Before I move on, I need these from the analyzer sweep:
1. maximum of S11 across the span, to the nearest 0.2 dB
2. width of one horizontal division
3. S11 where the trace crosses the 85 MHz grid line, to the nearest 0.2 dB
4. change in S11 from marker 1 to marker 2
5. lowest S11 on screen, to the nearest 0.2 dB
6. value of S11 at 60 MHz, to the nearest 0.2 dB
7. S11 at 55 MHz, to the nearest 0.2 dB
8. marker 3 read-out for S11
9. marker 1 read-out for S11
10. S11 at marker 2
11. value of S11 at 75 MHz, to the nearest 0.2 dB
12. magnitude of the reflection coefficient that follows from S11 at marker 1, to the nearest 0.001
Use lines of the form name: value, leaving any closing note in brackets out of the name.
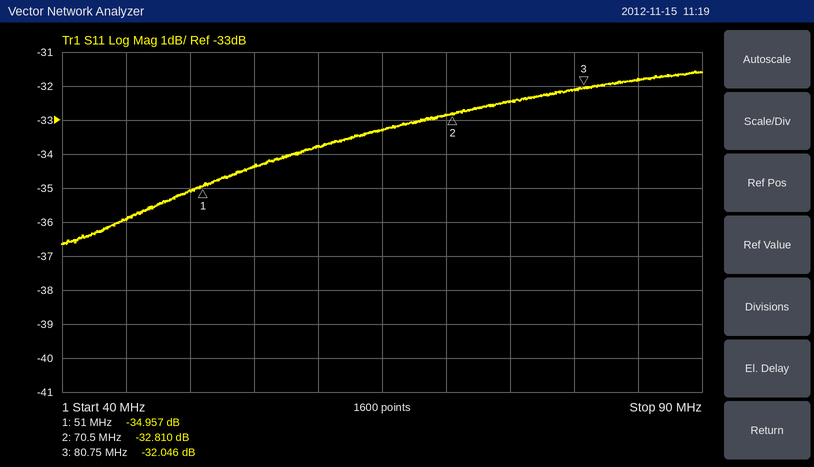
maximum of S11 across the span, to the nearest 0.2 dB: -31.6 dB
width of one horizontal division: 5 MHz
S11 where the trace crosses the 85 MHz grid line, to the nearest 0.2 dB: -31.8 dB
change in S11 from marker 1 to marker 2: 2.147 dB
lowest S11 on screen, to the nearest 0.2 dB: -36.6 dB
value of S11 at 60 MHz, to the nearest 0.2 dB: -33.8 dB
S11 at 55 MHz, to the nearest 0.2 dB: -34.4 dB
marker 3 read-out for S11: -32.046 dB
marker 1 read-out for S11: -34.957 dB
S11 at marker 2: -32.810 dB
value of S11 at 75 MHz, to the nearest 0.2 dB: -32.4 dB
magnitude of the reflection coefficient that follows from S11 at marker 1, to the nearest 0.001: 0.018
